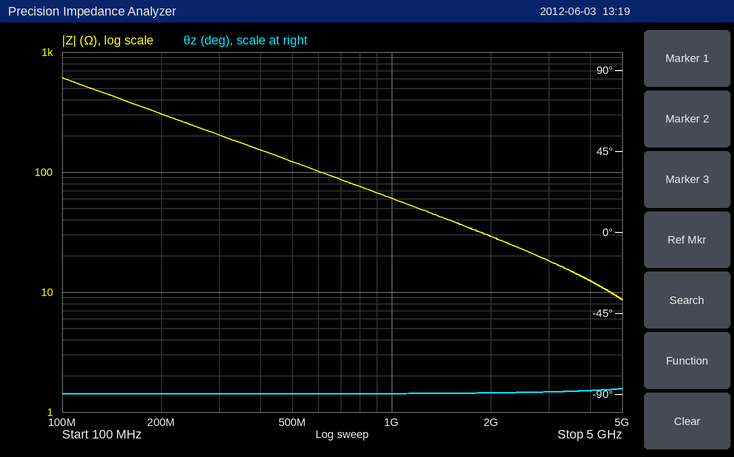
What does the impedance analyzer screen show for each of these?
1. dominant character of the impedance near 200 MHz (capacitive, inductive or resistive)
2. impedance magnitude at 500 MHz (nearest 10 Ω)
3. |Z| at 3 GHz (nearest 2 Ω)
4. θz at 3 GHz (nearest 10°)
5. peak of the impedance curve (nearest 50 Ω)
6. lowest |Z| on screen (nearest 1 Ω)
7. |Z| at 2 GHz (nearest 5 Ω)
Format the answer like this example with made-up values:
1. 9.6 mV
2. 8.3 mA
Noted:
1. capacitive
2. 120 Ω
3. 18 Ω
4. -90°
5. 600 Ω
6. 9 Ω
7. 30 Ω
